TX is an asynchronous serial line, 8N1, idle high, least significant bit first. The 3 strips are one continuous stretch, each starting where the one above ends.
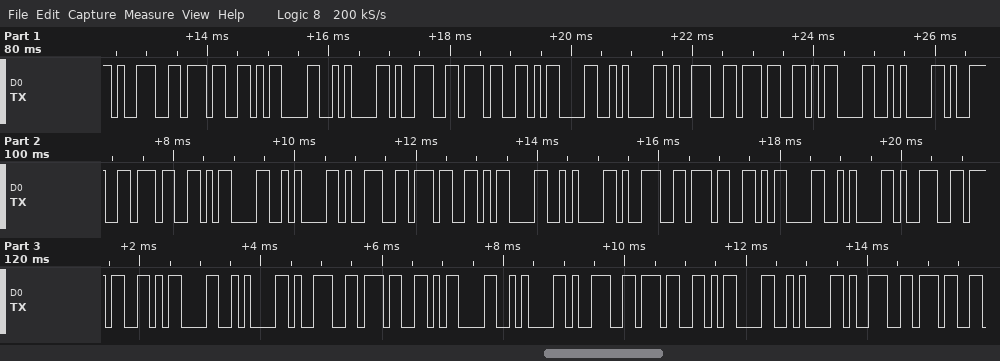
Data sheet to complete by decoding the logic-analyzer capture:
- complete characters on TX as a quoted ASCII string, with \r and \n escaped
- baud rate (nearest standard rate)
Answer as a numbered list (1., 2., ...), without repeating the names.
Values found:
1. "97\r\n97\r\n97\r\n97\r\n97\r\n97\r\n97\r\n97\r\n97\r\n97"
2. 9600 baud
